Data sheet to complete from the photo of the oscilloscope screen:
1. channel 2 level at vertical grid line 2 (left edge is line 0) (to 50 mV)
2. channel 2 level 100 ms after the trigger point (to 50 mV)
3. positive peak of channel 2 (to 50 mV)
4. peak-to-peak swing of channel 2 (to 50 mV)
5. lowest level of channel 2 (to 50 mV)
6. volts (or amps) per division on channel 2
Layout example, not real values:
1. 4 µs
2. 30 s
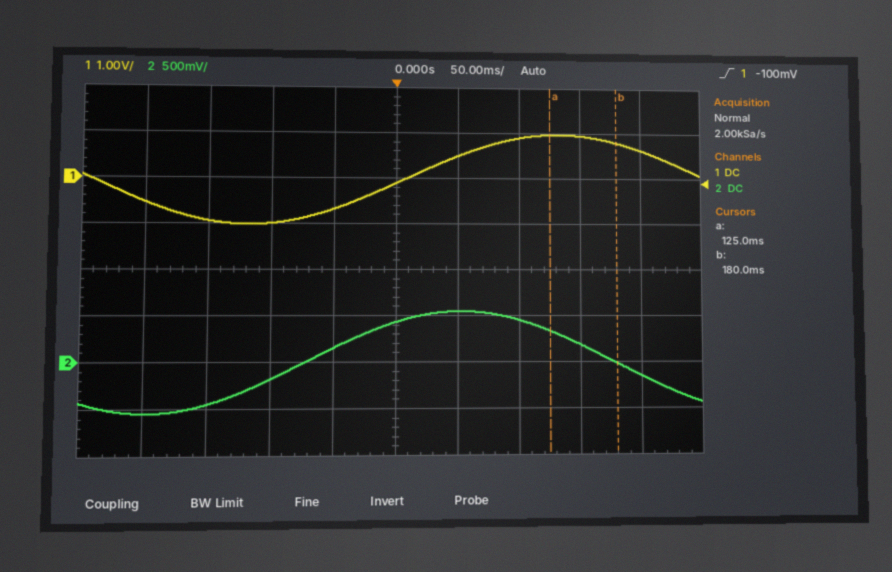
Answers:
1. -450 mV
2. 450 mV
3. 550 mV
4. 1.10 V
5. -550 mV
6. 500 mV
